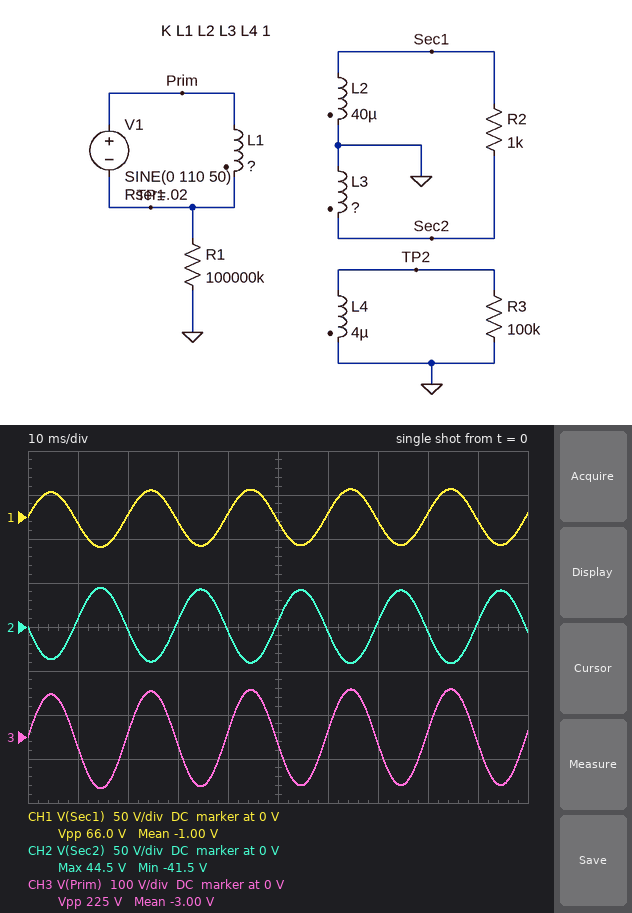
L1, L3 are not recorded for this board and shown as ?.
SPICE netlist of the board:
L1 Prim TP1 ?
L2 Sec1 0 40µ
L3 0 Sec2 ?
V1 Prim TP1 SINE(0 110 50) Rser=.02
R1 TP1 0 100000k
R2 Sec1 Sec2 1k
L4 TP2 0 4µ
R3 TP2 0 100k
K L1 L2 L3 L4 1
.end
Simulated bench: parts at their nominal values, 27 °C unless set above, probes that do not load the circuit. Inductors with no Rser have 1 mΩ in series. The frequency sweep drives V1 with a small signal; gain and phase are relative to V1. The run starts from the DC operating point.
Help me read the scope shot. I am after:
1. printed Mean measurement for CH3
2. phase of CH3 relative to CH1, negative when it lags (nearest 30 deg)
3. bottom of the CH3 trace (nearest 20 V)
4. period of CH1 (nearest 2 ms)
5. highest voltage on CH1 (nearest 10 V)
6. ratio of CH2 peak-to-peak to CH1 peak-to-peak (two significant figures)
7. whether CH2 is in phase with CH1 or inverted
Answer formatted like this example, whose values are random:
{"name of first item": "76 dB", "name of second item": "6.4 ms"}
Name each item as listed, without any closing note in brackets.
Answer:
{"printed Mean measurement for CH3": "-3.00 V", "phase of CH3 relative to CH1, negative when it lags": "0 deg", "bottom of the CH3 trace": "-120 V", "period of CH1": "20 ms", "highest voltage on CH1": "30 V", "ratio of CH2 peak-to-peak to CH1 peak-to-peak": "1.3", "whether CH2 is in phase with CH1 or inverted": "inverted"}
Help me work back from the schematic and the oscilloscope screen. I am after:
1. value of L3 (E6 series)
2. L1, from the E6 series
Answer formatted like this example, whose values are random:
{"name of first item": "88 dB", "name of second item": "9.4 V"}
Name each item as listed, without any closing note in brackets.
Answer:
{"value of L3": "68 µH", "L1, from the E6 series": "470 µH"}
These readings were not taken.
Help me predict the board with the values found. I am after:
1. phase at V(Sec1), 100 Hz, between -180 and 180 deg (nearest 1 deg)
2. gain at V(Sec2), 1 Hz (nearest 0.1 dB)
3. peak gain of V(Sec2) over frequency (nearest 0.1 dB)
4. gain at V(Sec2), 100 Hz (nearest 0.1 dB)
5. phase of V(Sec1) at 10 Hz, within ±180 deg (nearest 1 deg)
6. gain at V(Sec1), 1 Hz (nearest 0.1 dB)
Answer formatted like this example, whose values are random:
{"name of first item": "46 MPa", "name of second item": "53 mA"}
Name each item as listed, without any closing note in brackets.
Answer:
{"phase at V(Sec1), 100 Hz, between -180 and 180 deg": "4 deg", "gain at V(Sec2), 1 Hz": "-25.5 dB", "peak gain of V(Sec2) over frequency": "-8.4 dB", "gain at V(Sec2), 100 Hz": "-8.4 dB", "phase of V(Sec1) at 10 Hz, within ±180 deg": "35 deg", "gain at V(Sec1), 1 Hz": "-27.8 dB"}
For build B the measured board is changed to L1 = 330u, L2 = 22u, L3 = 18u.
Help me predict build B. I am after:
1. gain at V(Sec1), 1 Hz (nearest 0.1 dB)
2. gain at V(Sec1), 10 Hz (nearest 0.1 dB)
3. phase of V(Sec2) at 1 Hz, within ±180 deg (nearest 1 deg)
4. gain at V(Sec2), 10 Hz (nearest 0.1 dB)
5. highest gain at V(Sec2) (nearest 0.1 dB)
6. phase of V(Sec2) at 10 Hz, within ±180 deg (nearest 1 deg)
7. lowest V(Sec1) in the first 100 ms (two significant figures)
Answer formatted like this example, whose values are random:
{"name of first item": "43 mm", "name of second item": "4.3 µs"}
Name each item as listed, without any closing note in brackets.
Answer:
{"gain at V(Sec1), 1 Hz": "-31.9 dB", "gain at V(Sec1), 10 Hz": "-14.8 dB", "phase of V(Sec2) at 1 Hz, within ±180 deg": "-96 deg", "gain at V(Sec2), 10 Hz": "-15.7 dB", "highest gain at V(Sec2)": "-12.6 dB", "phase of V(Sec2) at 10 Hz, within ±180 deg": "-135 deg", "lowest V(Sec1) in the first 100 ms": "-30 V"}
